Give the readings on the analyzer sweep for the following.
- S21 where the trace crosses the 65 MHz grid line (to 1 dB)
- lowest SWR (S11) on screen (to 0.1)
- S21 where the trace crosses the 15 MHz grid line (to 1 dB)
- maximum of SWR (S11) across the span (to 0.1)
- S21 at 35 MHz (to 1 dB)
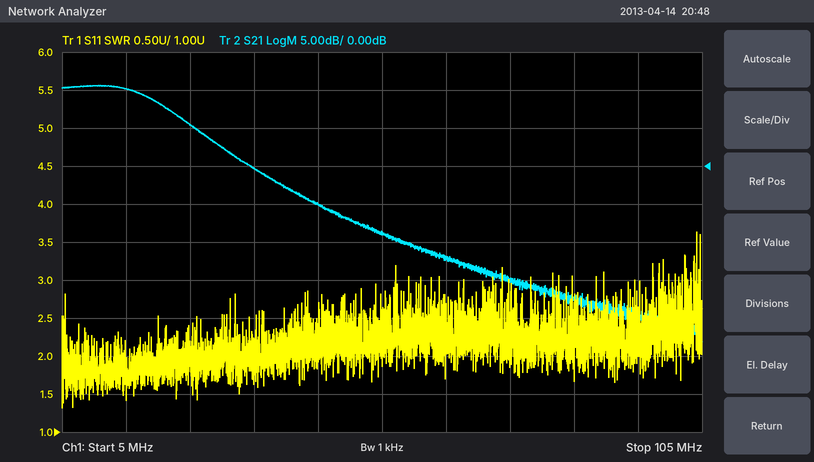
-12 dB
1.3
10 dB
3.6
0 dB
